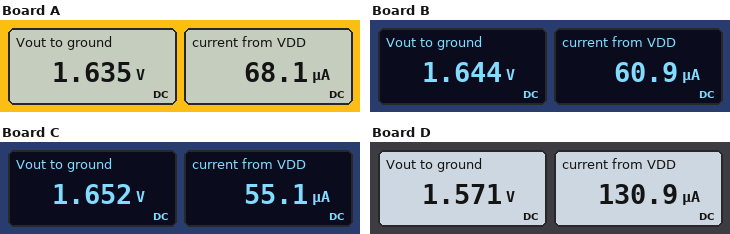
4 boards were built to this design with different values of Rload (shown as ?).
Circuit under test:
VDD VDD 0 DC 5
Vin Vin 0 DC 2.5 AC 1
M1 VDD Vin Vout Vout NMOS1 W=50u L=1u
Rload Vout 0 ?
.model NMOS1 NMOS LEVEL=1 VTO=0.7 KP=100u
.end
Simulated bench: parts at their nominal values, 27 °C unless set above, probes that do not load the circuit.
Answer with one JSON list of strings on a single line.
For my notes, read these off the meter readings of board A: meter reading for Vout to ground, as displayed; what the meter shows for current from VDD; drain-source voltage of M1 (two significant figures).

["1.635 V", "68.1 µA", "3.4 V"]
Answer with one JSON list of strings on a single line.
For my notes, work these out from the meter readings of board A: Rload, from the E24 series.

["24 kΩ"]
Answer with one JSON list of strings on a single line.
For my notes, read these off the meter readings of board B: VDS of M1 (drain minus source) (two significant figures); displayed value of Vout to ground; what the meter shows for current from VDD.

["3.4 V", "1.644 V", "60.9 µA"]
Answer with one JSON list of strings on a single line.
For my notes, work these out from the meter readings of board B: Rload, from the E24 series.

["27 kΩ"]
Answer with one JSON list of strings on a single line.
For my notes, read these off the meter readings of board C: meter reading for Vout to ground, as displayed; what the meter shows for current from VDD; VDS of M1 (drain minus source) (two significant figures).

["1.652 V", "55.1 µA", "3.3 V"]
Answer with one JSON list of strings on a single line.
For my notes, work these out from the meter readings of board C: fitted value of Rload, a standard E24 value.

["30 kΩ"]
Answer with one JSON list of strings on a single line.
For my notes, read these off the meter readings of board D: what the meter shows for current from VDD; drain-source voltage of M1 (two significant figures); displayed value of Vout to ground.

["130.9 µA", "3.4 V", "1.571 V"]
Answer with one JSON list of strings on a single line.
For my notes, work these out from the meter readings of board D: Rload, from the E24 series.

["12 kΩ"]
